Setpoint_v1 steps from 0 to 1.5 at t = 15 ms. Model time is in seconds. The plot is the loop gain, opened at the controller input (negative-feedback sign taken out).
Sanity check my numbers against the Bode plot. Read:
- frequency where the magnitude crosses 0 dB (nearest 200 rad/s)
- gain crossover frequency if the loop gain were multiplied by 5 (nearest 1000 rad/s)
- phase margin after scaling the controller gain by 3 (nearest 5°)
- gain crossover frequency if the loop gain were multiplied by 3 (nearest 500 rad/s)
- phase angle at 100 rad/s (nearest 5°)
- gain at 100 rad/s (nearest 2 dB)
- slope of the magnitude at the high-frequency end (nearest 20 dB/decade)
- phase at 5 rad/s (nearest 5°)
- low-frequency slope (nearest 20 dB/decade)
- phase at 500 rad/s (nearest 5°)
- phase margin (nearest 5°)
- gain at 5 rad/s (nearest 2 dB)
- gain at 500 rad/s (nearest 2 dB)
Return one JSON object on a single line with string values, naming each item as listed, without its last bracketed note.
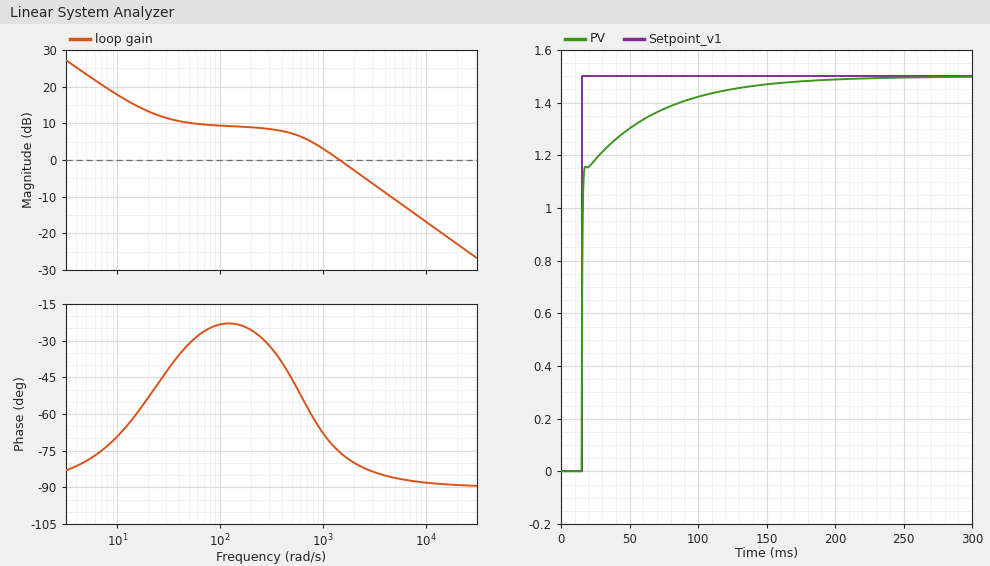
{"frequency where the magnitude crosses 0 dB": "1400 rad/s", "gain crossover frequency if the loop gain were multiplied by 5": "7000 rad/s", "phase margin after scaling the controller gain by 3": "95°", "gain crossover frequency if the loop gain were multiplied by 3": "4500 rad/s", "phase angle at 100 rad/s": "-25°", "gain at 100 rad/s": "10 dB", "slope of the magnitude at the high-frequency end": "-20 dB/decade", "phase at 5 rad/s": "-80°", "low-frequency slope": "-20 dB/decade", "phase at 500 rad/s": "-45°", "phase margin": "105°", "gain at 5 rad/s": "24 dB", "gain at 500 rad/s": "8 dB"}
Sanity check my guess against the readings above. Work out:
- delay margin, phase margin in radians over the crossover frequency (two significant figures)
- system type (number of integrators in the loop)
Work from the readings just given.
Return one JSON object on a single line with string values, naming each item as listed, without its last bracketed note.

{"delay margin, phase margin in radians over the crossover frequency": "0.0013 s", "system type": "1"}
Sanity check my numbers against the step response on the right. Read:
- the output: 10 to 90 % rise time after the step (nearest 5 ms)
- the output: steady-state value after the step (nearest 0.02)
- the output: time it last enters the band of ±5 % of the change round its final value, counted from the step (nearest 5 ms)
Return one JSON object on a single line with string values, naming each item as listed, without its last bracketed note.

{"the output: 10 to 90 % rise time after the step": "50 ms", "the output: steady-state value after the step": "1.50", "the output: time it last enters the band of ±5 % of the change round its final value, counted from the step": "85 ms"}
